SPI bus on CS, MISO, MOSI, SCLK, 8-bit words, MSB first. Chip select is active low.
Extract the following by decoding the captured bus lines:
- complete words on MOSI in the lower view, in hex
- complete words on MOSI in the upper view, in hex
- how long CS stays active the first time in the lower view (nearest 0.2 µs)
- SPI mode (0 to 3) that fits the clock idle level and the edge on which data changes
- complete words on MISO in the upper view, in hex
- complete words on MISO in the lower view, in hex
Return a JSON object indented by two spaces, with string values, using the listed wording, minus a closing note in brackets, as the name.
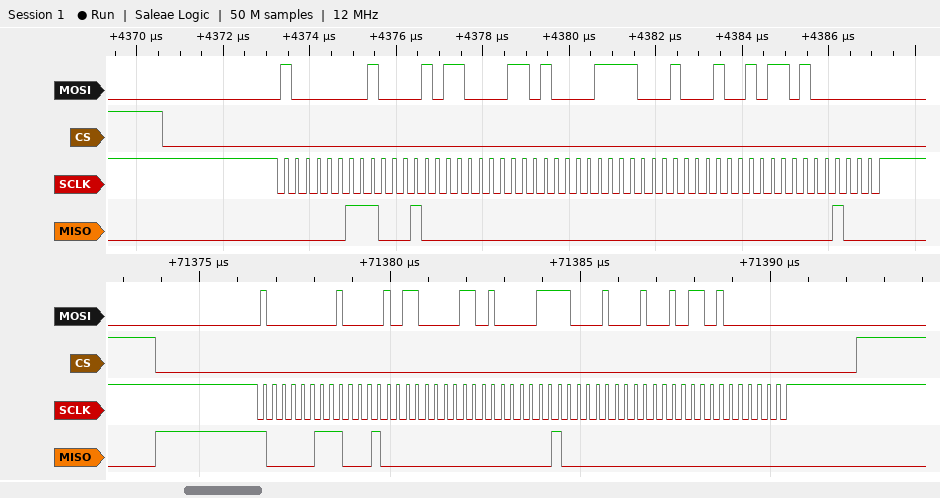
{
  "complete words on MOSI in the lower view, in hex": "80, 85, 86, 87, 88, 96, 80",
  "complete words on MOSI in the upper view, in hex": "80, 85, 86, 87, 88, 96, 80",
  "how long CS stays active the first time in the lower view": "18.4 µs",
  "SPI mode (0 to 3) that fits the clock idle level and the edge on which data changes": "3",
  "complete words on MISO in the upper view, in hex": "03, 88, 00, 00, 00, 00, 10",
  "complete words on MISO in the lower view, in hex": "83, 88, 00, 01, 00, 00, 00"
}
